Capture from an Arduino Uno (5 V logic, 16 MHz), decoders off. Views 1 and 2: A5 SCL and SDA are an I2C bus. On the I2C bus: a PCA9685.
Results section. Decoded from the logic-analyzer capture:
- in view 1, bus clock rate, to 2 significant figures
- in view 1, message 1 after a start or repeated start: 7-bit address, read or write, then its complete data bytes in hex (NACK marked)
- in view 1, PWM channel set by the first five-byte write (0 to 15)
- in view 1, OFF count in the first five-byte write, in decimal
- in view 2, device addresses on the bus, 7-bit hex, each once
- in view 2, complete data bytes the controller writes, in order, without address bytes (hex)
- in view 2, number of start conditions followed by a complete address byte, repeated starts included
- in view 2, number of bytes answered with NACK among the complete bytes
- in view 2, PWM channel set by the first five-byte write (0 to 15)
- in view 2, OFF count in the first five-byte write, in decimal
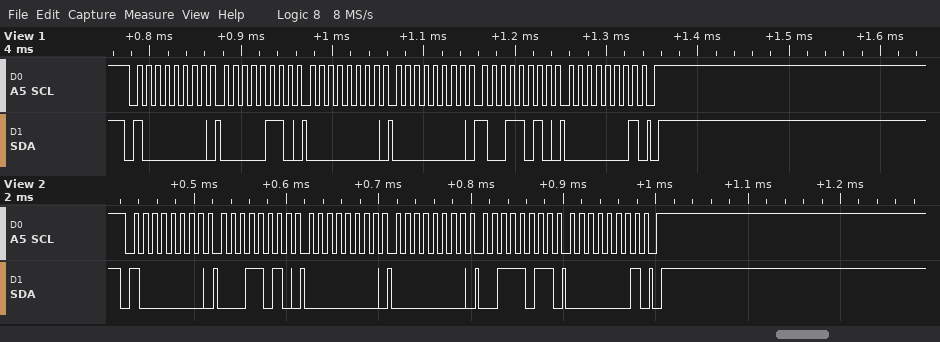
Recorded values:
100 kHz
0x40 write: 06 00 00 9A 01
0
410
0x40
1A 00 00 3B 01
1
0
5
315
